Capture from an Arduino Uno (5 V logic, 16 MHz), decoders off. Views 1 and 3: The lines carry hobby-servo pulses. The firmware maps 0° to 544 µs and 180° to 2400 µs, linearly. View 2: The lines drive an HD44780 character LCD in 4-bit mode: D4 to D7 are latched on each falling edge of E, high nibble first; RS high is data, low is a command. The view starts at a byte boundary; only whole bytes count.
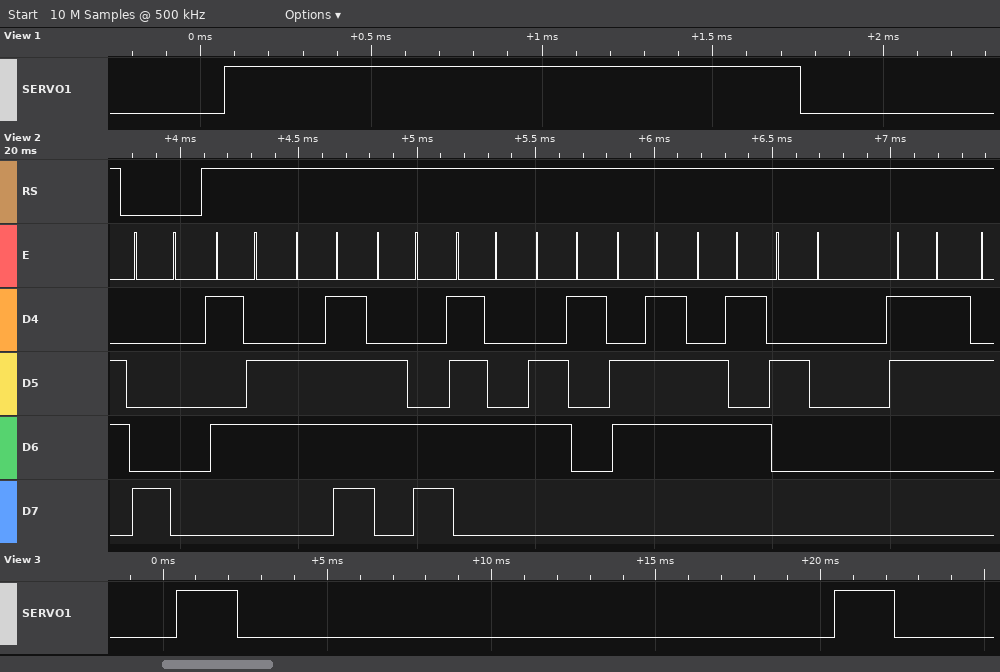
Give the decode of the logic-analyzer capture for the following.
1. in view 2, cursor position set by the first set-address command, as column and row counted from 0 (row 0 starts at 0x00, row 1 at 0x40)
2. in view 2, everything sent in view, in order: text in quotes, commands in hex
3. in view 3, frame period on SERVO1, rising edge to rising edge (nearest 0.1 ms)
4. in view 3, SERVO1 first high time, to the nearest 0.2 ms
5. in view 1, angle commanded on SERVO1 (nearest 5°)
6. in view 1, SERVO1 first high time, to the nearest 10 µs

column 0, row 0
0x80 "Voltage 3"
20.0 ms
1.8 ms
110°
1690 µs
